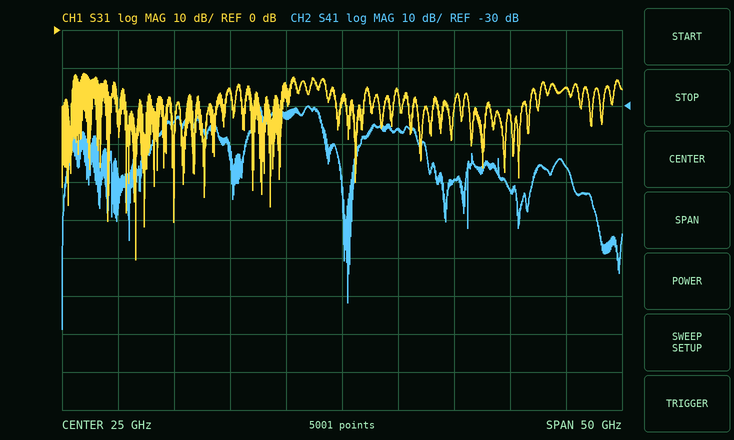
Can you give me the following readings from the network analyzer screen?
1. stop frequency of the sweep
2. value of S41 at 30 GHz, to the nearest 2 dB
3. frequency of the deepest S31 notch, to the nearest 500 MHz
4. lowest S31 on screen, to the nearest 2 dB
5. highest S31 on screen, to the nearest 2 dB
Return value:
50 GHz
-36 dB
6.5 GHz
-60 dB
-12 dB
